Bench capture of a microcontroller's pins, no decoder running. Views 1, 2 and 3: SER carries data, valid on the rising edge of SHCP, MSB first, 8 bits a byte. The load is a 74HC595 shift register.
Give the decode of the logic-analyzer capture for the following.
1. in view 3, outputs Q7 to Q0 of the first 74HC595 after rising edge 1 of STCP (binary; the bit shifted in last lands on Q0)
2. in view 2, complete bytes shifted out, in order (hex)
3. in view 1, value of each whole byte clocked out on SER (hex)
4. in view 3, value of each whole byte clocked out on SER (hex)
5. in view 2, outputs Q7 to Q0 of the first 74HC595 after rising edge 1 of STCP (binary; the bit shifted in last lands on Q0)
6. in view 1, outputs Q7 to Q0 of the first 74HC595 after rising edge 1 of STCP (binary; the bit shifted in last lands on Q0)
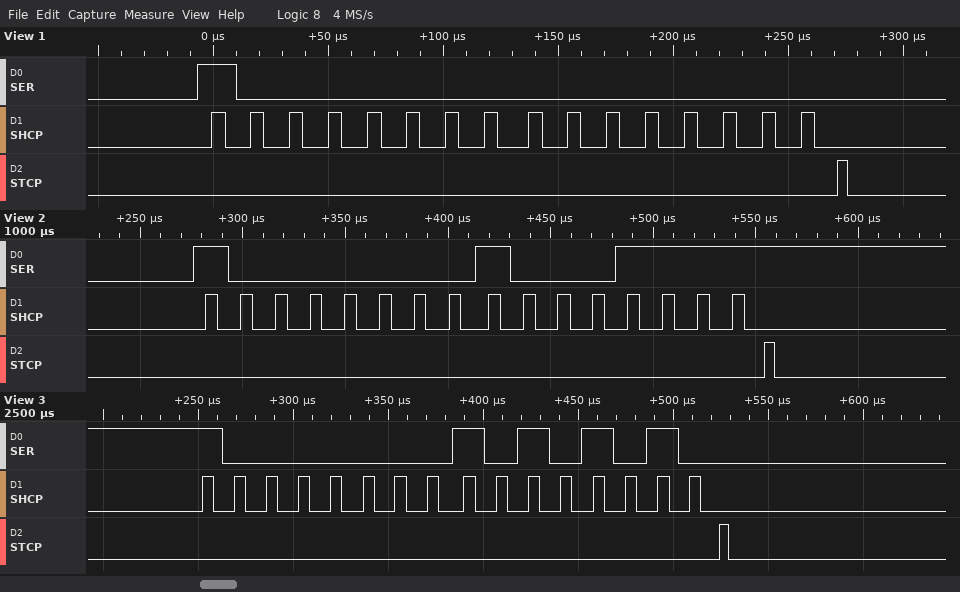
10101010
80 8F
0x80 0x00
80 AA
10001111
00000000
